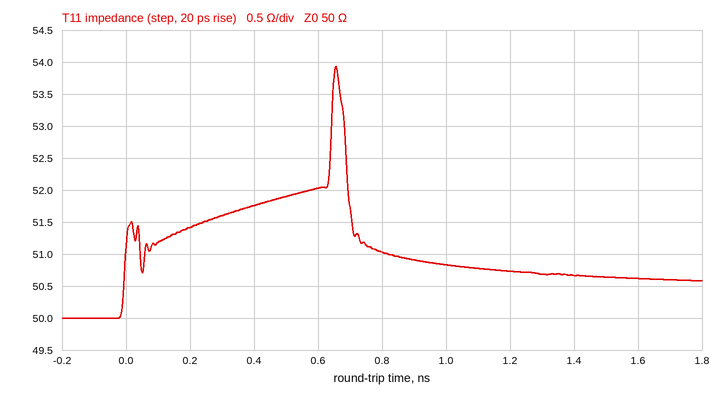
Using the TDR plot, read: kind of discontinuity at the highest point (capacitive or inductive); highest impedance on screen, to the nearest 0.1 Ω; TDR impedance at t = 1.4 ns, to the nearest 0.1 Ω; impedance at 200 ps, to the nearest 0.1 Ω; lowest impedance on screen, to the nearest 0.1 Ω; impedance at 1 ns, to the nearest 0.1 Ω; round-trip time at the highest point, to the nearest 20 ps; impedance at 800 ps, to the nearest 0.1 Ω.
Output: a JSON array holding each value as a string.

["inductive", "53.9 Ω", "50.7 Ω", "51.4 Ω", "50.0 Ω", "50.8 Ω", "660 ps", "51.0 Ω"]
